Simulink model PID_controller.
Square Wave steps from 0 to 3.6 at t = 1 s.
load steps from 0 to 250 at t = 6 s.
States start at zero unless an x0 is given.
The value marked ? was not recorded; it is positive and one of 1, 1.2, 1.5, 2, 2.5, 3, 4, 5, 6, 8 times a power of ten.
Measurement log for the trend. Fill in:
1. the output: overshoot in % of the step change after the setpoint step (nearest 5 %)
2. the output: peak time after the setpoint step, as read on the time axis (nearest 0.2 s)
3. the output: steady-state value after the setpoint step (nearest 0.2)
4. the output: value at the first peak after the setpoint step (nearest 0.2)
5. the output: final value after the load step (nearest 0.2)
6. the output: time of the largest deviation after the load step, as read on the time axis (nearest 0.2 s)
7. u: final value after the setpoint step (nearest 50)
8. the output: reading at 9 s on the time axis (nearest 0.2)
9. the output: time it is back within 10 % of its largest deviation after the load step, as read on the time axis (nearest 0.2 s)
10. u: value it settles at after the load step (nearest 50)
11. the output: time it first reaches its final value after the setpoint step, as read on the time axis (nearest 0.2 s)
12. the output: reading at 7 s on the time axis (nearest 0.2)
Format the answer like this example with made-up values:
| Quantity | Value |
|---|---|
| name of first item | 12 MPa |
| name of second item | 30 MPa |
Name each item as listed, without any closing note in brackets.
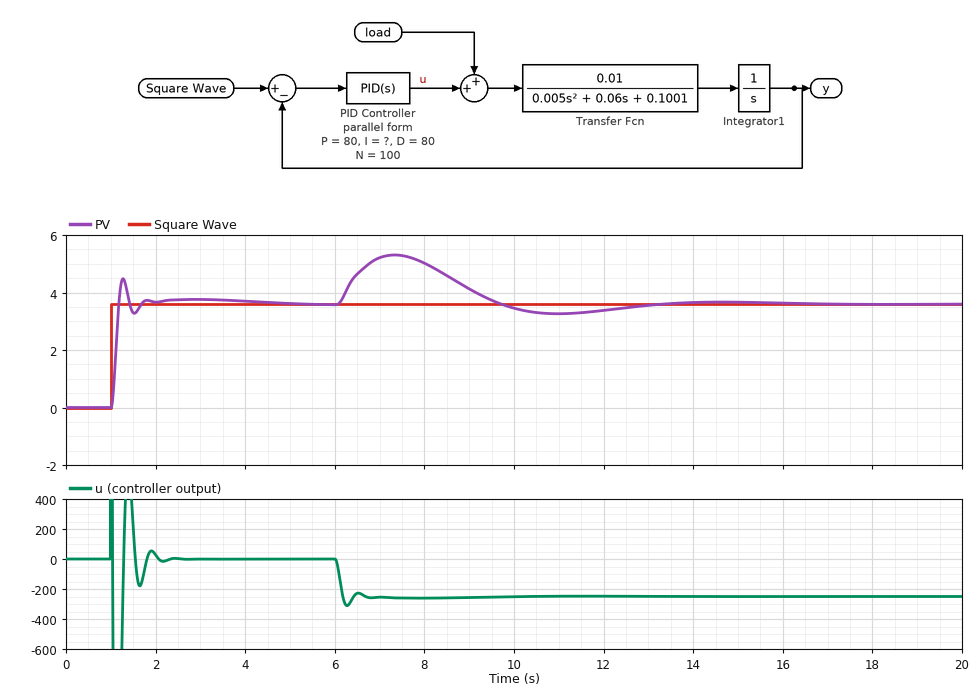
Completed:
| Quantity | Value |
|---|---|
| the output: overshoot in % of the step change after the setpoint step | 25 % |
| the output: peak time after the setpoint step, as read on the time axis | 1.2 s |
| the output: steady-state value after the setpoint step | 3.6 |
| the output: value at the first peak after the setpoint step | 4.4 |
| the output: final value after the load step | 3.6 |
| the output: time of the largest deviation after the load step, as read on the time axis | 7.4 s |
| u: final value after the setpoint step | 0 |
| the output: reading at 9 s on the time axis | 4.2 |
| the output: time it is back within 10 % of its largest deviation after the load step, as read on the time axis | 12.2 s |
| u: value it settles at after the load step | -250 |
| the output: time it first reaches its final value after the setpoint step, as read on the time axis | 1.2 s |
| the output: reading at 7 s on the time axis | 5.2 |
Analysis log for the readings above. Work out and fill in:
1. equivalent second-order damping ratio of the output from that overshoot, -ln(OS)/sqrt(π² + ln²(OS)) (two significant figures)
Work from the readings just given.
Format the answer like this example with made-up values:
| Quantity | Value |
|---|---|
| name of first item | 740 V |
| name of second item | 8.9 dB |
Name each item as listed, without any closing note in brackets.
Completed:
| Quantity | Value |
|---|---|
| equivalent second-order damping ratio of the output from that overshoot, -ln(OS)/sqrt(π² + ln²(OS)) | 0.40 |
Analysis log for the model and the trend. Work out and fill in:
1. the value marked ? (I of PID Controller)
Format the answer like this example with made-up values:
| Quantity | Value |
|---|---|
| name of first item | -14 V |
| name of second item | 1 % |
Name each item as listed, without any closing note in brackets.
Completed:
| Quantity | Value |
|---|---|
| the value marked ? | 80 |
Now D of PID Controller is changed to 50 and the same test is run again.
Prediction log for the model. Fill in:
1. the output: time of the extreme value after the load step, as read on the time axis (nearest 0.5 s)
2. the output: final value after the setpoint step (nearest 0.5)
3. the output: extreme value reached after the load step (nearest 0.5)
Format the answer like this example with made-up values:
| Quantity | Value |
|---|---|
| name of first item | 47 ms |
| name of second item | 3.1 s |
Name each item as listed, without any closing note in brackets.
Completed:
| Quantity | Value |
|---|---|
| the output: time of the extreme value after the load step, as read on the time axis | 7.0 s |
| the output: final value after the setpoint step | 3.5 |
| the output: extreme value reached after the load step | 5.5 |
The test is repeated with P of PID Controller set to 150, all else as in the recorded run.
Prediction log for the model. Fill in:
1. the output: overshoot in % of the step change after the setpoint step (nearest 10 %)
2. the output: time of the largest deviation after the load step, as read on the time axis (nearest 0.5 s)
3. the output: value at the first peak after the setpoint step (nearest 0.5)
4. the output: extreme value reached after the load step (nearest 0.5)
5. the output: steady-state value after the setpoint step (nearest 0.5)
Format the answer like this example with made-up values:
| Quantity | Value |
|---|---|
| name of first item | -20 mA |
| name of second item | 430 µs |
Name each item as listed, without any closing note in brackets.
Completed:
| Quantity | Value |
|---|---|
| the output: overshoot in % of the step change after the setpoint step | 30 % |
| the output: time of the largest deviation after the load step, as read on the time axis | 7.0 s |
| the output: value at the first peak after the setpoint step | 5.0 |
| the output: extreme value reached after the load step | 5.0 |
| the output: steady-state value after the setpoint step | 3.5 |
